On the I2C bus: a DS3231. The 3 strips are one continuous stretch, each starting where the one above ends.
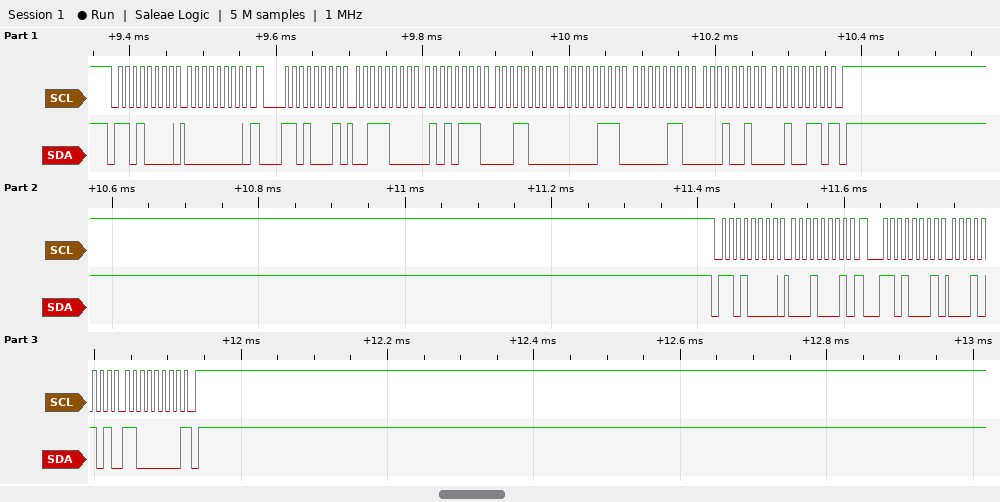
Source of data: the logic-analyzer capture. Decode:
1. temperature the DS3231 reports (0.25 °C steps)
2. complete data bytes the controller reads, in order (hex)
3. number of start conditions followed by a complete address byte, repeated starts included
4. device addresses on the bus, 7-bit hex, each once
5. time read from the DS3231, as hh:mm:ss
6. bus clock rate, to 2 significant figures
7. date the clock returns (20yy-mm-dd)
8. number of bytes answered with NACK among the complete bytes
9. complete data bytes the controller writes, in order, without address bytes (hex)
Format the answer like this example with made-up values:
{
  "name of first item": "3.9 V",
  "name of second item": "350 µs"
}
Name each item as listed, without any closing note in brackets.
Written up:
{
  "temperature the DS3231 reports": "21.75 °C",
  "complete data bytes the controller reads, in order": "38 57 18 07 06 12 26 15 C0",
  "number of start conditions followed by a complete address byte, repeated starts included": "4",
  "device addresses on the bus, 7-bit hex, each once": "0x68",
  "time read from the DS3231, as hh:mm:ss": "18:57:38",
  "bus clock rate, to 2 significant figures": "100 kHz",
  "date the clock returns": "2026-12-06",
  "number of bytes answered with NACK among the complete bytes": "2",
  "complete data bytes the controller writes, in order, without address bytes": "00 11"
}
